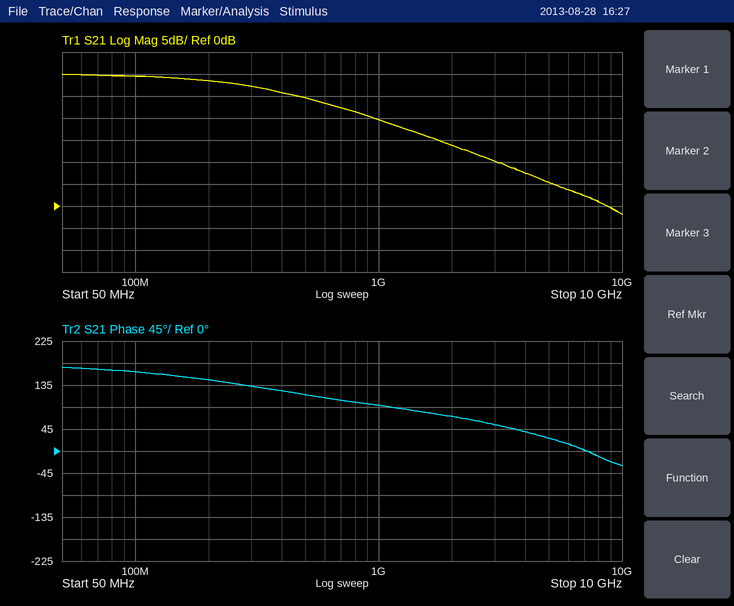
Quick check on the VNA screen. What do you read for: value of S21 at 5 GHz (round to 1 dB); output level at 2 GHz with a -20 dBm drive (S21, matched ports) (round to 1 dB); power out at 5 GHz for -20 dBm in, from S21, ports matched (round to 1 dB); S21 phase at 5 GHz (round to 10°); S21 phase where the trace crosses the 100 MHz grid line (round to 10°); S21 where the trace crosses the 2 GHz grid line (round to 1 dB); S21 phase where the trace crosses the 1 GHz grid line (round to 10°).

5 dB
-6 dBm
-15 dBm
30°
160°
14 dB
90°
